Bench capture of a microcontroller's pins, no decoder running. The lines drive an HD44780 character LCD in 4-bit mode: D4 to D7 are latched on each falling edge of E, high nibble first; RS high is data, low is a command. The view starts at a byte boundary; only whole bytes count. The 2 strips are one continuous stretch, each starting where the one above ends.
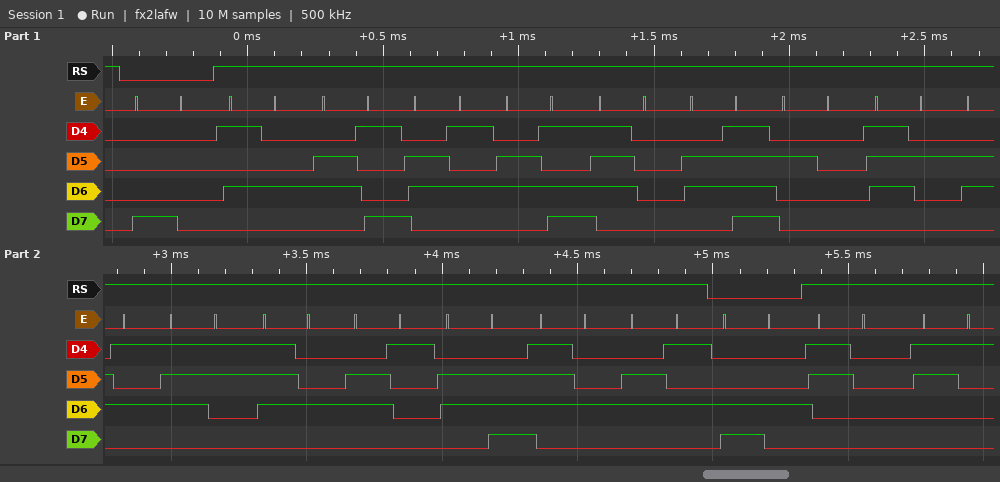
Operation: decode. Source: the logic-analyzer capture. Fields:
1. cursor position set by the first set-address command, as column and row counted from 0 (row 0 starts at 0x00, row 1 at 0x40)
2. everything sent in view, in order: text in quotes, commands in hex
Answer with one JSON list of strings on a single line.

["column 0, row 0", "0x80 \"Tiempo restante\" 0xC4 \"01\""]
